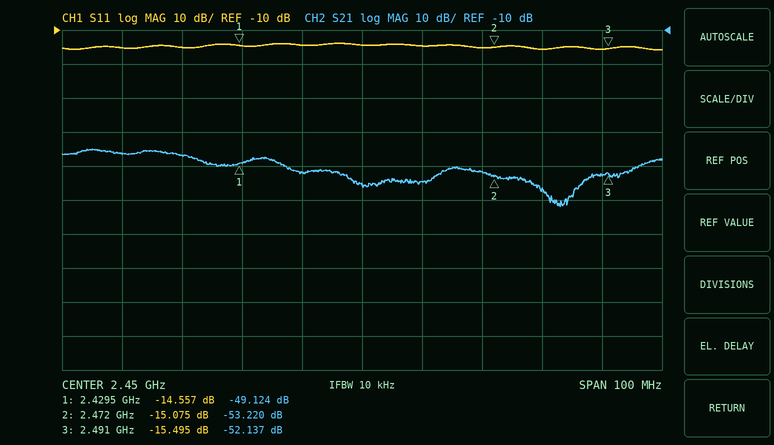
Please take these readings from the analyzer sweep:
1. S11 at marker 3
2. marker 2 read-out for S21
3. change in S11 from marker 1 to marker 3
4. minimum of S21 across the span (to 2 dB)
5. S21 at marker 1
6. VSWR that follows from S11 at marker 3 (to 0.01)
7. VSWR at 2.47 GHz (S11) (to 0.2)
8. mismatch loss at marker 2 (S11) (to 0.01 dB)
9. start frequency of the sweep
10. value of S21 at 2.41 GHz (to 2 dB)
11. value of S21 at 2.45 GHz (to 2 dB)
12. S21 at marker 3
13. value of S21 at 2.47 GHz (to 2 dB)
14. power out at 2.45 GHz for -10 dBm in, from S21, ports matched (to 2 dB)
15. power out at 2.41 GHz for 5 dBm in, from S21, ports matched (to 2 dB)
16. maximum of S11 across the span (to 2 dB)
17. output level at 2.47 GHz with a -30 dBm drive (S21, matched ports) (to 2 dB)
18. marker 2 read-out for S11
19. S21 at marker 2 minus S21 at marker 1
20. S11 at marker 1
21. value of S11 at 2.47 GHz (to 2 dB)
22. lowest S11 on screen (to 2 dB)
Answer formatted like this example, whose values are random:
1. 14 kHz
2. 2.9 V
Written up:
1. -15.495 dB
2. -53.220 dB
3. -0.938 dB
4. -62 dB
5. -49.124 dB
6. 1.40
7. 1.4
8. 0.14 dB
9. 2.4 GHz
10. -46 dB
11. -56 dB
12. -52.137 dB
13. -52 dB
14. -66 dBm
15. -42 dBm
16. -14 dB
17. -82 dBm
18. -15.075 dB
19. -4.096 dB
20. -14.557 dB
21. -16 dB
22. -16 dB
